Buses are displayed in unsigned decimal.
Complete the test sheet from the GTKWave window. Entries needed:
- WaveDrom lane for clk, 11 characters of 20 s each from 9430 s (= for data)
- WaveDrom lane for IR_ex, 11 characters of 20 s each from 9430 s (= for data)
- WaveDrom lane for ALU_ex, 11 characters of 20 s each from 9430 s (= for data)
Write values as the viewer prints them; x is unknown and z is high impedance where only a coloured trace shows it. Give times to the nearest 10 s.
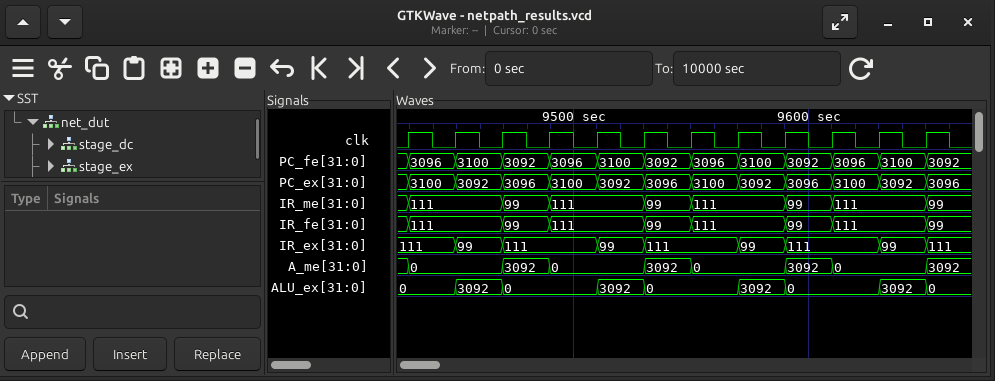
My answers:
{name: 'clk', wave: 'p..........'}
{name: 'IR_ex', wave: '===.==.==.=', data: '111 99 111 99 111 99 111 99'}
{name: 'ALU_ex', wave: '===.==.==.=', data: '0 3092 0 3092 0 3092 0 3092'}
